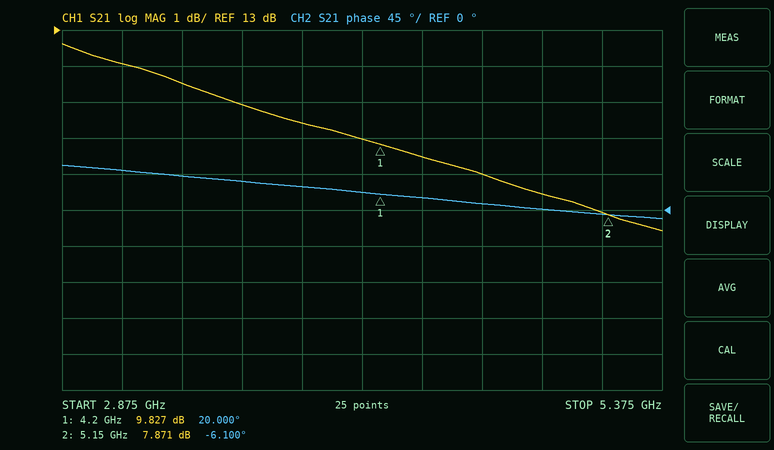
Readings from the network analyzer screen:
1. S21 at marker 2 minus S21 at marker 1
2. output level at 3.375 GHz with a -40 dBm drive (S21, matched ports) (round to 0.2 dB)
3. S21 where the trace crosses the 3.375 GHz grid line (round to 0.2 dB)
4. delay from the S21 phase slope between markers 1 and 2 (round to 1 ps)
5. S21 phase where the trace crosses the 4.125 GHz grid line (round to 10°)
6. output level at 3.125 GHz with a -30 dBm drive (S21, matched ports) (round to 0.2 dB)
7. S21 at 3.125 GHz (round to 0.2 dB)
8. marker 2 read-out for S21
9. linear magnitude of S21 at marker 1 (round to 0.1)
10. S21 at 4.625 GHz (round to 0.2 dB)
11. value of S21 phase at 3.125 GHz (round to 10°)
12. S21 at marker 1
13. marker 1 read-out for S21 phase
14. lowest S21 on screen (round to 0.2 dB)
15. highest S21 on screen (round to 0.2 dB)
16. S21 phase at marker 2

-1.956 dB
-28.4 dBm
11.6 dB
76 ps
20°
-18.0 dBm
12.0 dB
7.871 dB
3.1
9.0 dB
50°
9.827 dB
20.000°
7.4 dB
12.6 dB
-6.100°
